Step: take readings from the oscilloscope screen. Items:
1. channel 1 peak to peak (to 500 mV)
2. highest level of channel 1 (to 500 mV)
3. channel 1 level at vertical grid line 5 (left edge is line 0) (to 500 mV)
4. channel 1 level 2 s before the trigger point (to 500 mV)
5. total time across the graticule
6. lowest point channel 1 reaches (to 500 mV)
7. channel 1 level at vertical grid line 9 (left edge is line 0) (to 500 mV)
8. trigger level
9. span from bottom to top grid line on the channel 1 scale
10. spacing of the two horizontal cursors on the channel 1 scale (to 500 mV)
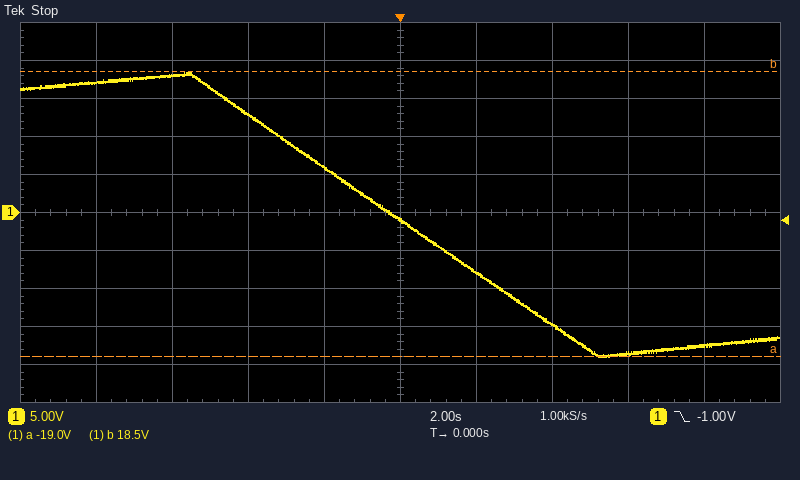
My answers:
37.5 V
18.5 V
-1.0 V
6.0 V
20 s
-19.0 V
-17.5 V
-1.00 V
50 V
37.5 V
